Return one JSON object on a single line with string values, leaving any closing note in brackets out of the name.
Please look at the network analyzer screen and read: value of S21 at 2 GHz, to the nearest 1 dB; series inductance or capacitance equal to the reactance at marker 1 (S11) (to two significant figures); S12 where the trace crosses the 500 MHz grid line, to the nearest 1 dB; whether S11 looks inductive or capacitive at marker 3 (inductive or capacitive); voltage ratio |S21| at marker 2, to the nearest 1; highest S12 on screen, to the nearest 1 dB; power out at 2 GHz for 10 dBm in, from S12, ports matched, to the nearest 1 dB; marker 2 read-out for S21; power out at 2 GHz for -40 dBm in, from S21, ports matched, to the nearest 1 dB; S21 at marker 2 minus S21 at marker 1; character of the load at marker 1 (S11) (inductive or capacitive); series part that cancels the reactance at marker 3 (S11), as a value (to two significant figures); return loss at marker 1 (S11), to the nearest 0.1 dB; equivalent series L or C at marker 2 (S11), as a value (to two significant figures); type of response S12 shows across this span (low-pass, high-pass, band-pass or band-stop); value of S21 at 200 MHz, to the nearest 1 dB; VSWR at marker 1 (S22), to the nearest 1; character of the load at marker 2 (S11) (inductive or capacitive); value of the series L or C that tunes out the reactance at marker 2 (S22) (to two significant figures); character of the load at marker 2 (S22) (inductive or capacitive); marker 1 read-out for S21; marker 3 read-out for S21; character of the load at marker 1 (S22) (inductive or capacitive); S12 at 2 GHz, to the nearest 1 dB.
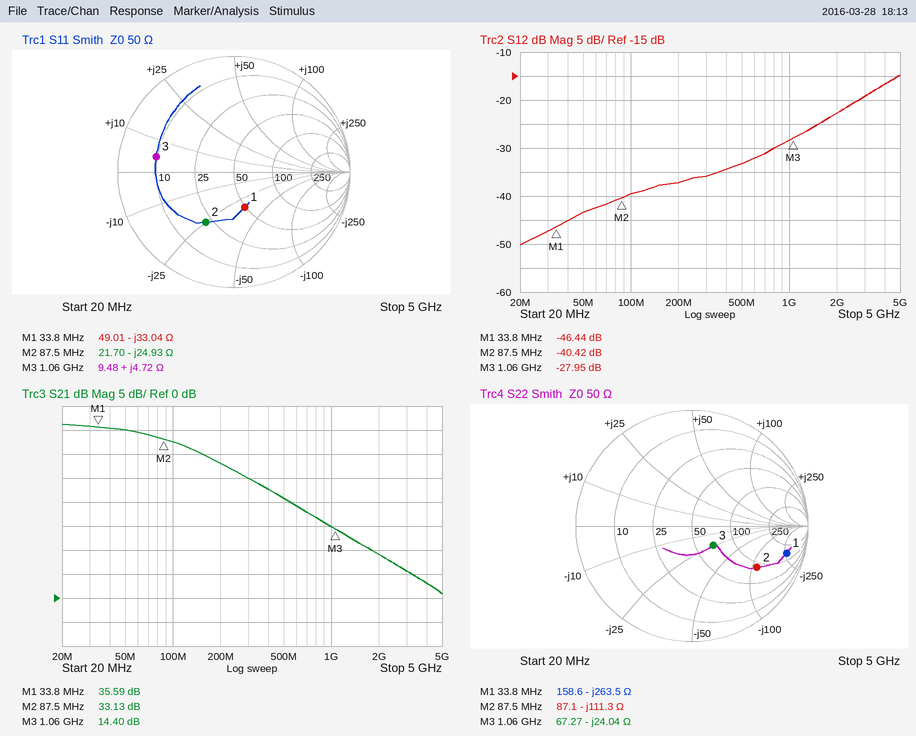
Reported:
{"value of S21 at 2 GHz, to the nearest 1 dB": "9 dB", "series inductance or capacitance equal to the reactance at marker 1 (S11)": "140 pF", "S12 where the trace crosses the 500 MHz grid line, to the nearest 1 dB": "-33 dB", "whether S11 looks inductive or capacitive at marker 3": "inductive", "voltage ratio |S21| at marker 2, to the nearest 1": "45", "highest S12 on screen, to the nearest 1 dB": "-15 dB", "power out at 2 GHz for 10 dBm in, from S12, ports matched, to the nearest 1 dB": "-13 dBm", "marker 2 read-out for S21": "33.13 dB", "power out at 2 GHz for -40 dBm in, from S21, ports matched, to the nearest 1 dB": "-31 dBm", "S21 at marker 2 minus S21 at marker 1": "-2.46 dB", "character of the load at marker 1 (S11)": "capacitive", "series part that cancels the reactance at marker 3 (S11), as a value": "32 pF", "return loss at marker 1 (S11), to the nearest 0.1 dB": "10.0 dB", "equivalent series L or C at marker 2 (S11), as a value": "73 pF", "type of response S12 shows across this span": "high-pass", "value of S21 at 200 MHz, to the nearest 1 dB": "28 dB", "VSWR at marker 1 (S22), to the nearest 1": "12", "character of the load at marker 2 (S11)": "capacitive", "value of the series L or C that tunes out the reactance at marker 2 (S22)": "200 nH", "character of the load at marker 2 (S22)": "capacitive", "marker 1 read-out for S21": "35.59 dB", "marker 3 read-out for S21": "14.40 dB", "character of the load at marker 1 (S22)": "capacitive", "S12 at 2 GHz, to the nearest 1 dB": "-23 dB"}
